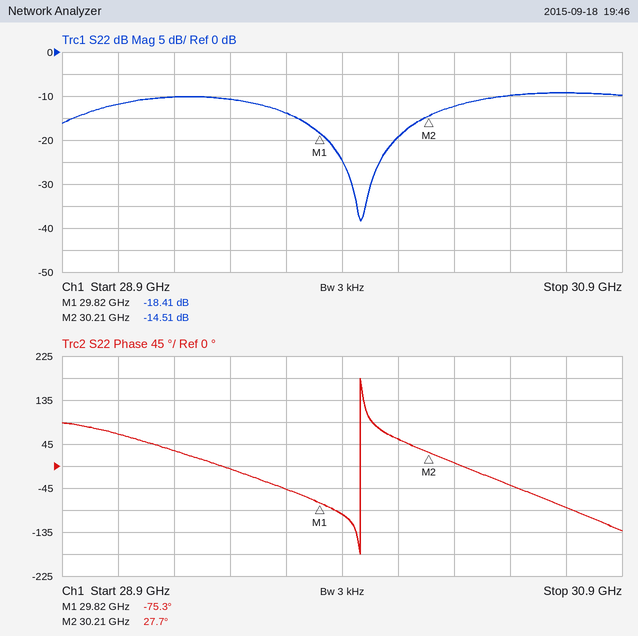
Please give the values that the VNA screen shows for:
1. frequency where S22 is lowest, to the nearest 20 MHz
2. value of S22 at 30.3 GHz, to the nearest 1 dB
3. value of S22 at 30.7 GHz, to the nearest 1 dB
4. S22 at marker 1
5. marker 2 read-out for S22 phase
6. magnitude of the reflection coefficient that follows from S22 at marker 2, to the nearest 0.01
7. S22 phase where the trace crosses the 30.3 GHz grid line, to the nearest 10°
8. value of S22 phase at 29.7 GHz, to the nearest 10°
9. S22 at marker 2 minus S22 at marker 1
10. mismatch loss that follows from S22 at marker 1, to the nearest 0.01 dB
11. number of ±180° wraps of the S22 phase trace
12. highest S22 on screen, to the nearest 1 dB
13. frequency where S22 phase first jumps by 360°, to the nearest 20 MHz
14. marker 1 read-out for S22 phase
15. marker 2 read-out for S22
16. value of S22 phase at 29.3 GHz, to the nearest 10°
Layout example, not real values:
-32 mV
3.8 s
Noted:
29.96 GHz
-12 dB
-9 dB
-18.41 dB
27.7°
0.19
10°
-50°
3.90 dB
0.06 dB
1
-9 dB
29.96 GHz
-75.3°
-14.51 dB
30°
